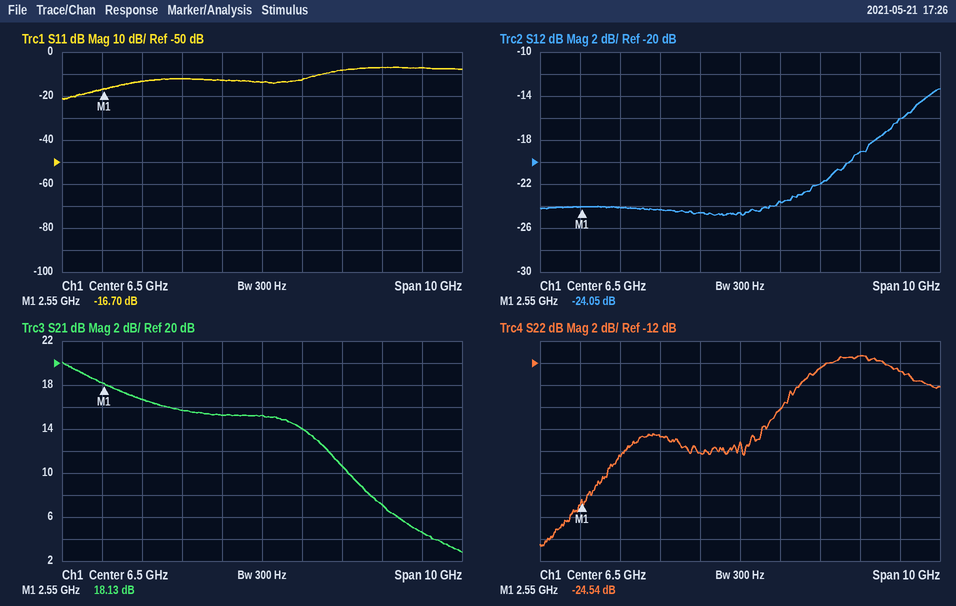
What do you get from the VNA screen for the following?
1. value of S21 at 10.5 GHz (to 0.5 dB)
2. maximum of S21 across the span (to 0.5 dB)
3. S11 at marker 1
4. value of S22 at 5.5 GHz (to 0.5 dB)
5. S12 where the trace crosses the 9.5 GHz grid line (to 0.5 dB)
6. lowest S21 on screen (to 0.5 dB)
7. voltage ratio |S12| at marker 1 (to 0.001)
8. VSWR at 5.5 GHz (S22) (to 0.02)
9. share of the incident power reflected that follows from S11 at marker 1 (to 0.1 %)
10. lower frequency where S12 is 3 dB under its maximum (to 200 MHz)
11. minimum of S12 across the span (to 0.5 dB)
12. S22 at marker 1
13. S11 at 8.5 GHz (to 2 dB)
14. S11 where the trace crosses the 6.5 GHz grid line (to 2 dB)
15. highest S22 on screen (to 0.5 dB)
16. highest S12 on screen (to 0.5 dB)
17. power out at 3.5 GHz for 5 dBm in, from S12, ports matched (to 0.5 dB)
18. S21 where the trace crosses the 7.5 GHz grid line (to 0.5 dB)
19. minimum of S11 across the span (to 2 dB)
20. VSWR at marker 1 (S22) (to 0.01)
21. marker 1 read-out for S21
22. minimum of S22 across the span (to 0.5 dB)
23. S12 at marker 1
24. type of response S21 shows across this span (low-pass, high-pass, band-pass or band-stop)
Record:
4.5 dB
20.0 dB
-16.70 dB
-20.0 dB
-19.0 dB
3.0 dB
0.063
1.22
2.1 %
10.4 GHz
-25.0 dB
-24.54 dB
-8 dB
-14 dB
-11.5 dB
-13.5 dB
-19.0 dBm
14.0 dB
-22 dB
1.13
18.13 dB
-28.5 dB
-24.05 dB
low-pass
